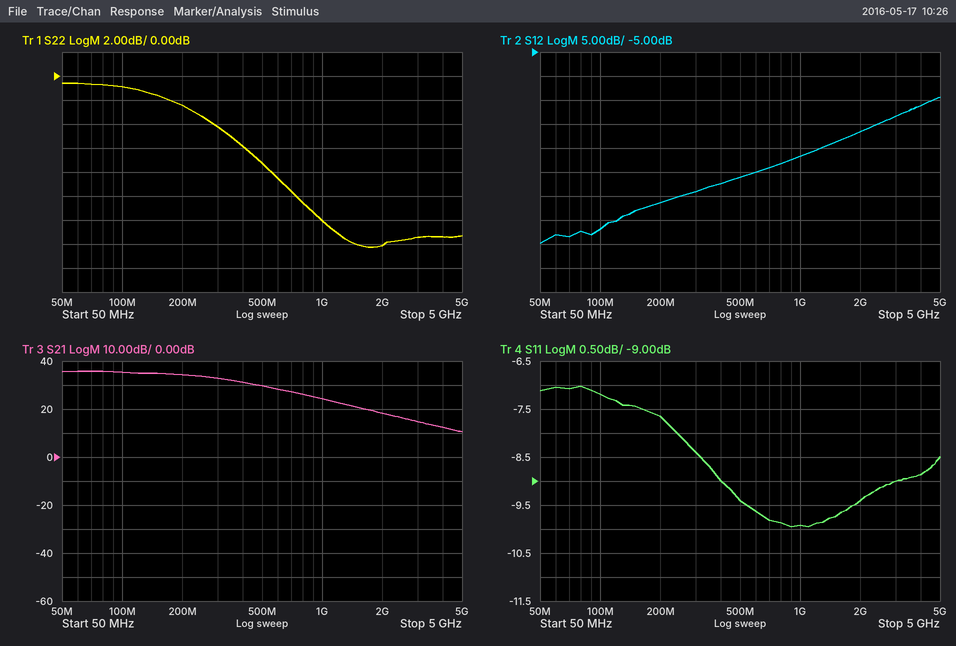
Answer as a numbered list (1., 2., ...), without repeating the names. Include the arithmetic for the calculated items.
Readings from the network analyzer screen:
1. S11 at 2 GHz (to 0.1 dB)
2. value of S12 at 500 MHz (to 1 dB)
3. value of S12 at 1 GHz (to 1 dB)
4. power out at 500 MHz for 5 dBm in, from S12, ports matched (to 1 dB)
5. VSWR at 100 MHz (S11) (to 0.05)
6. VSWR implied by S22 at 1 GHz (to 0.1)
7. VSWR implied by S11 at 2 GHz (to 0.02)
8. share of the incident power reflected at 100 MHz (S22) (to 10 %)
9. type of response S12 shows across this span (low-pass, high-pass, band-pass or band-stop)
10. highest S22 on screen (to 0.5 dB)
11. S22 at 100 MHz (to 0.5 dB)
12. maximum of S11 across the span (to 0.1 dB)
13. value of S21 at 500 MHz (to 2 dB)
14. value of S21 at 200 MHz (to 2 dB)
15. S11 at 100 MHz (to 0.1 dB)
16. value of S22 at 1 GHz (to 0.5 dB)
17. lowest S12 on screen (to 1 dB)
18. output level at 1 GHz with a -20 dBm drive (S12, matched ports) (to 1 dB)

1. -9.4 dB
2. -31 dB
3. -27 dB
4. 5 dBm + (-31 dB) = -26 dBm
5. |Γ| = 10^(-7.2/20) = 0.4365; VSWR = (1 + 0.4365)/(1 − 0.4365) ≈ 2.55
6. |Γ| = 10^(-12/20) = 0.2512; VSWR = (1 + 0.2512)/(1 − 0.2512) ≈ 1.7
7. |Γ| = 10^(-9.4/20) = 0.3388; VSWR = (1 + 0.3388)/(1 − 0.3388) ≈ 2.03, so 2.02 to the nearest 0.02
8. 10^(-1/10) ≈ 79.4 %, so 80 % to the nearest 10 %
9. high-pass
10. -0.5 dB
11. -1.0 dB
12. -7.0 dB
13. 30 dB
14. 34 dB
15. -7.2 dB
16. -12.0 dB
17. -45 dB
18. -20 dBm + (-27 dB) = -47 dBm
